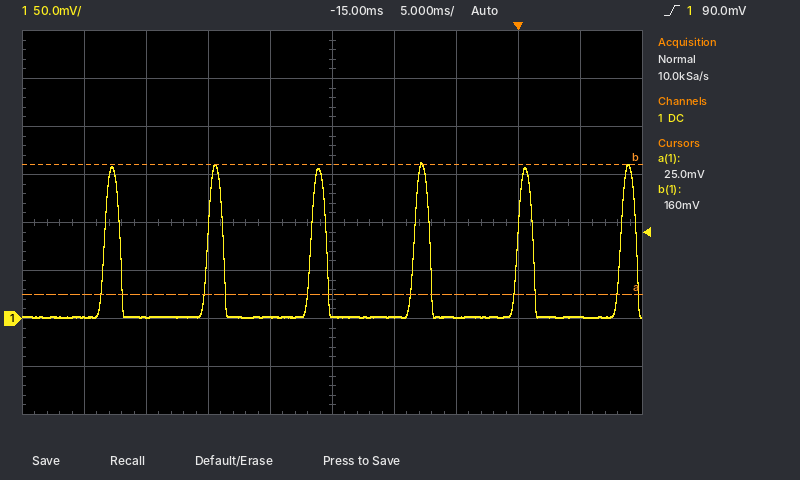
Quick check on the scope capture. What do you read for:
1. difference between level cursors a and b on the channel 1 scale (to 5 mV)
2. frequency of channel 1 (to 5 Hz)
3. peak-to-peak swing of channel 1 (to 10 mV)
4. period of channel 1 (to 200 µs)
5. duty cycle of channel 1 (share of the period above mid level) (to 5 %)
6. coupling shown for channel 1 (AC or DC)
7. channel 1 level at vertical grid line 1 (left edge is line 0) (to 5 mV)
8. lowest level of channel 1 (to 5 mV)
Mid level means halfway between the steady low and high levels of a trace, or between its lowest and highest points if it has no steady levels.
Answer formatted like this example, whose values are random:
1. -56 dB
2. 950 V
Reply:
1. 135 mV
2. 120 Hz
3. 160 mV
4. 8.4 ms
5. 15 %
6. DC
7. 0 mV
8. 0 mV
